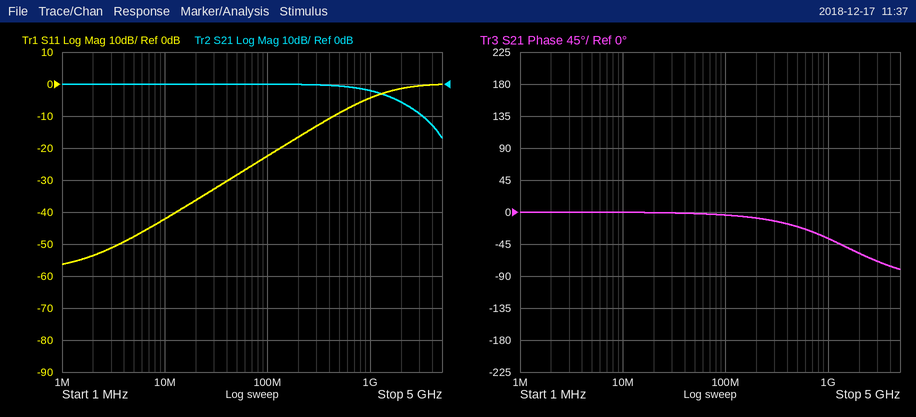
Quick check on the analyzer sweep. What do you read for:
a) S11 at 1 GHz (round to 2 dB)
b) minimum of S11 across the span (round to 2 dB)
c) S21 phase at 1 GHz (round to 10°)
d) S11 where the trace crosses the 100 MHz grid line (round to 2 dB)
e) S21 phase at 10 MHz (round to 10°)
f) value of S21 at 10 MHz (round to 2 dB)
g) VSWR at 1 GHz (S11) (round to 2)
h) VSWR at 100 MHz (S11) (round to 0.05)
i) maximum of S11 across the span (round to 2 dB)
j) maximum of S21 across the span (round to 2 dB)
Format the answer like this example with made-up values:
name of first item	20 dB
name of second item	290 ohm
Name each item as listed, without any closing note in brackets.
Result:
S11 at 1 GHz	-4 dB
minimum of S11 across the span	-56 dB
S21 phase at 1 GHz	-40°
S11 where the trace crosses the 100 MHz grid line	-22 dB
S21 phase at 10 MHz	0°
value of S21 at 10 MHz	0 dB
VSWR at 1 GHz (S11)	4
VSWR at 100 MHz (S11)	1.15
maximum of S11 across the span	0 dB
maximum of S21 across the span	0 dB
